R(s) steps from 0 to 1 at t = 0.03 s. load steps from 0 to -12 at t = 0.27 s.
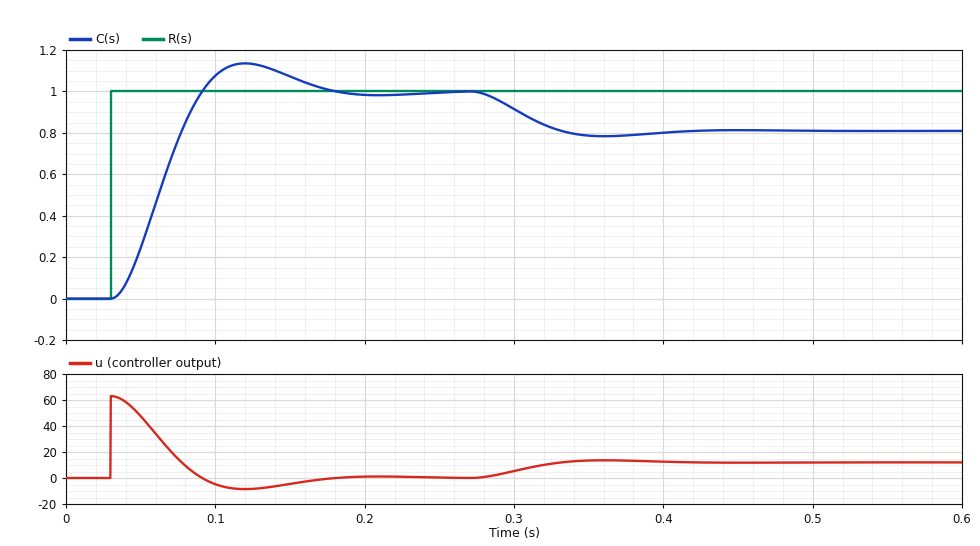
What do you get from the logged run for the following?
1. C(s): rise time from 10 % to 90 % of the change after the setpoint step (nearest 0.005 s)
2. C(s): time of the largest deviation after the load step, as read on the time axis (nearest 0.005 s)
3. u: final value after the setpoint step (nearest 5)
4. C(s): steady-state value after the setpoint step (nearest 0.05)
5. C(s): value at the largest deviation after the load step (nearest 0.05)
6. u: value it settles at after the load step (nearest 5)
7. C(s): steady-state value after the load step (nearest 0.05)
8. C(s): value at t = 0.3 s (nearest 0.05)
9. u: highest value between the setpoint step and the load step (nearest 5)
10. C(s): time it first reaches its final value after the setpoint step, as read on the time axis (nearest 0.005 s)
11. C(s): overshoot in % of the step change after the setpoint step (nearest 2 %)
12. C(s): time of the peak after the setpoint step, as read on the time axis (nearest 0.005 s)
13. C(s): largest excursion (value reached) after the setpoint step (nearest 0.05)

0.040 s
0.360 s
0
1.00
0.80
10
0.80
0.90
65
0.090 s
14 %
0.120 s
1.15
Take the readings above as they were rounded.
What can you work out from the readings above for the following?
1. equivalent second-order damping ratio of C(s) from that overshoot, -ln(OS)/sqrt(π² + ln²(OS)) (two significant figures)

0.53
